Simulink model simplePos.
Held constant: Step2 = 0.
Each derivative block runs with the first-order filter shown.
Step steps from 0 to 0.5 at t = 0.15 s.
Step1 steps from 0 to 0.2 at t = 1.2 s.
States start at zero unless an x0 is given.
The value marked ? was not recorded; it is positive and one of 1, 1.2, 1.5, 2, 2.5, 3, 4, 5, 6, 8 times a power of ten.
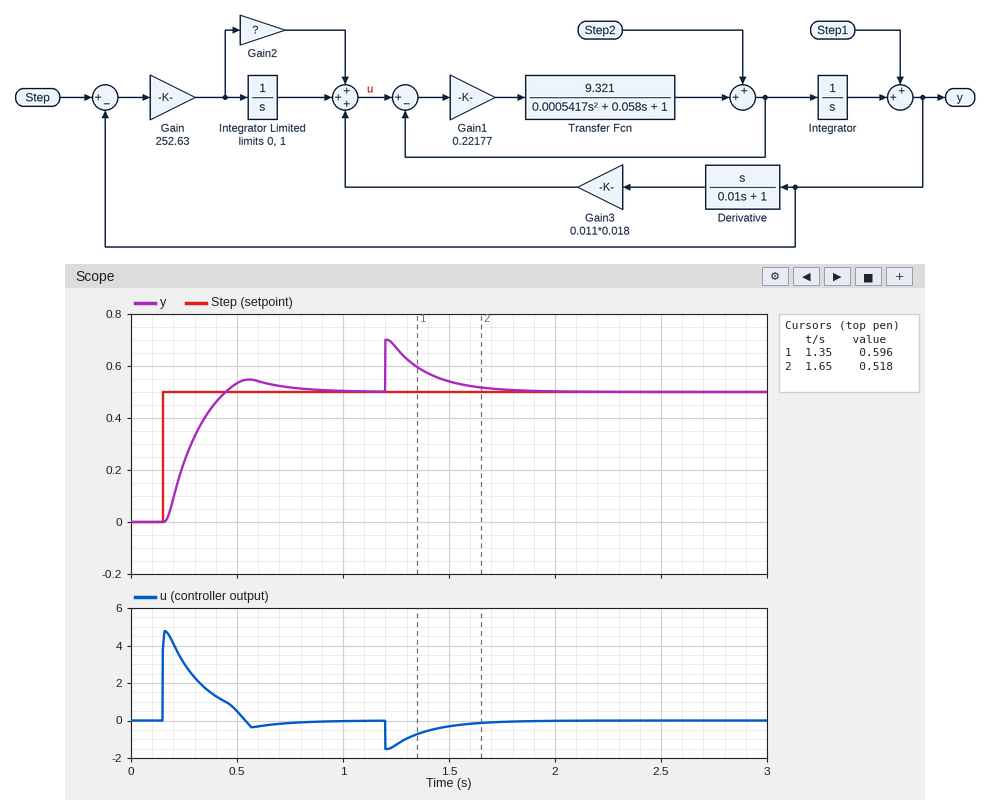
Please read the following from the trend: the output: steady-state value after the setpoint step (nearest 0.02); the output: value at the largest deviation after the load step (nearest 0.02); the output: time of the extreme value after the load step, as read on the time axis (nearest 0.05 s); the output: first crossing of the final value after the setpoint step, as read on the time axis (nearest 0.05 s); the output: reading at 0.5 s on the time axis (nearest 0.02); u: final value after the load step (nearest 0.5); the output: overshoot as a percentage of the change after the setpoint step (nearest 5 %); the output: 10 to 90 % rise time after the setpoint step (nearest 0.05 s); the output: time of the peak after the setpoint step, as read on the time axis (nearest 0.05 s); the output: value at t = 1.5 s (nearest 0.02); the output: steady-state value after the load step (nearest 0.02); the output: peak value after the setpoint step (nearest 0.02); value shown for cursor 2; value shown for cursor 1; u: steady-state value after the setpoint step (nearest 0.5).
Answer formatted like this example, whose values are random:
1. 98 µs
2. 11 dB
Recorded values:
1. 0.50
2. 0.70
3. 1.20 s
4. 0.45 s
5. 0.54
6. 0.0
7. 10 %
8. 0.20 s
9. 0.55 s
10. 0.54
11. 0.50
12. 0.54
13. 0.518
14. 0.596
15. 0.0
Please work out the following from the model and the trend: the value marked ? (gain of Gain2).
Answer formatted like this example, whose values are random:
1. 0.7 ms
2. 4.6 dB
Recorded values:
1. 0.03
